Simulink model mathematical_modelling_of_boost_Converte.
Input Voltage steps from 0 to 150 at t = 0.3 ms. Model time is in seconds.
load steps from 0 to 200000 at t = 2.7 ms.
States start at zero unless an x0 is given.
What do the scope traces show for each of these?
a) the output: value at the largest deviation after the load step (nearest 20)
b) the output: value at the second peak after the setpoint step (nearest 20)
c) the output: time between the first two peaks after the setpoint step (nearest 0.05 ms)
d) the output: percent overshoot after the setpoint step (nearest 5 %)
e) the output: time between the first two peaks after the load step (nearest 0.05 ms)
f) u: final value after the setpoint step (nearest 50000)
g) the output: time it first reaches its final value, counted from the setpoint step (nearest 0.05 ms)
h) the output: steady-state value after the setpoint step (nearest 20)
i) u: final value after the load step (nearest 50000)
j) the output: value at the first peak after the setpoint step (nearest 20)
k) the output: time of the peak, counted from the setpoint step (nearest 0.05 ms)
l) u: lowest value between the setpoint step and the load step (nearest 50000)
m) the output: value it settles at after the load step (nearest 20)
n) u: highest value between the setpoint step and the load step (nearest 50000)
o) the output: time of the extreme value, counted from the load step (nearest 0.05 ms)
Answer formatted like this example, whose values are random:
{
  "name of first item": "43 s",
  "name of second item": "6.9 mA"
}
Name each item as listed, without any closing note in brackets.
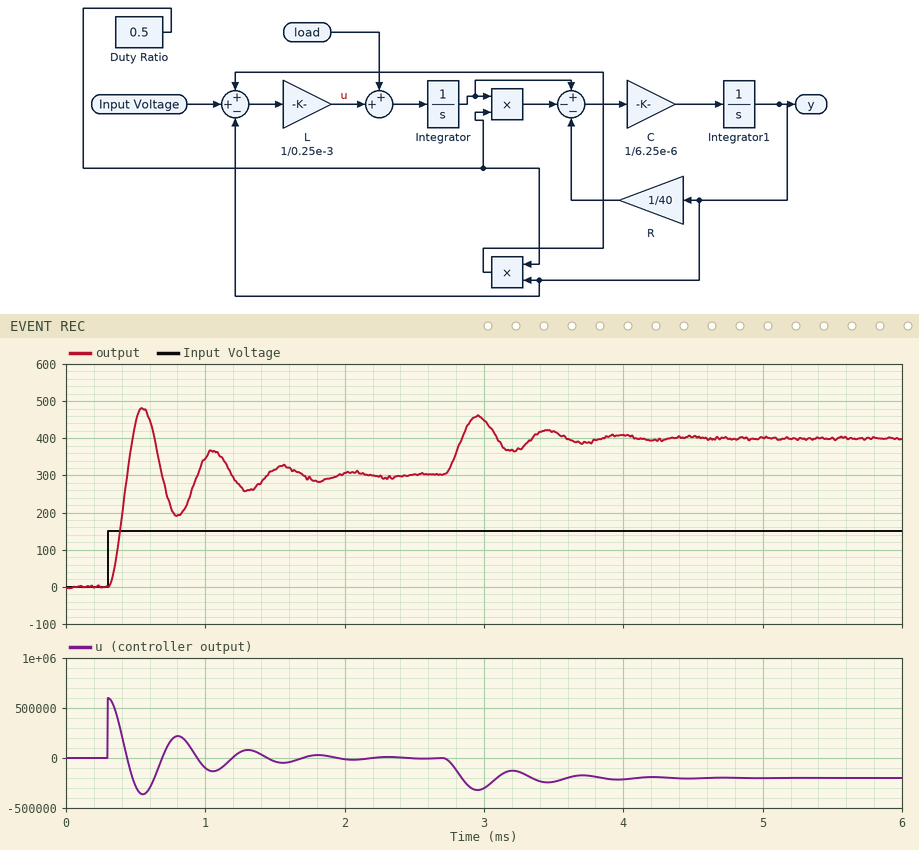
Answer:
{
  "the output: value at the largest deviation after the load step": "460",
  "the output: value at the second peak after the setpoint step": "360",
  "the output: time between the first two peaks after the setpoint step": "0.50 ms",
  "the output: percent overshoot after the setpoint step": "60 %",
  "the output: time between the first two peaks after the load step": "0.50 ms",
  "u: final value after the setpoint step": "0",
  "the output: time it first reaches its final value, counted from the setpoint step": "0.15 ms",
  "the output: steady-state value after the setpoint step": "300",
  "u: final value after the load step": "-200000",
  "the output: value at the first peak after the setpoint step": "480",
  "the output: time of the peak, counted from the setpoint step": "0.25 ms",
  "u: lowest value between the setpoint step and the load step": "-350000",
  "the output: value it settles at after the load step": "400",
  "u: highest value between the setpoint step and the load step": "600000",
  "the output: time of the extreme value, counted from the load step": "0.25 ms"
}
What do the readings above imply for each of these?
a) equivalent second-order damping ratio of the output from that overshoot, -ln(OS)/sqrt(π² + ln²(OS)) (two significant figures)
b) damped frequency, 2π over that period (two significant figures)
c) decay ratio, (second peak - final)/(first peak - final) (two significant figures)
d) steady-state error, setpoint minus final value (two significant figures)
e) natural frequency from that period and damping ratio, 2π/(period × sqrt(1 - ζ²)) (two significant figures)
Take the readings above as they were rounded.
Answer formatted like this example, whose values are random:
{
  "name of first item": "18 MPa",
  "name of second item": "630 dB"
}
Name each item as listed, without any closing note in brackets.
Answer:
{
  "equivalent second-order damping ratio of the output from that overshoot, -ln(OS)/sqrt(π² + ln²(OS))": "0.16",
  "damped frequency, 2π over that period": "13 rad/ms",
  "decay ratio, (second peak - final)/(first peak - final)": "0.33",
  "steady-state error, setpoint minus final value": "-150",
  "natural frequency from that period and damping ratio, 2π/(period × sqrt(1 - ζ²))": "13 rad/ms"
}
